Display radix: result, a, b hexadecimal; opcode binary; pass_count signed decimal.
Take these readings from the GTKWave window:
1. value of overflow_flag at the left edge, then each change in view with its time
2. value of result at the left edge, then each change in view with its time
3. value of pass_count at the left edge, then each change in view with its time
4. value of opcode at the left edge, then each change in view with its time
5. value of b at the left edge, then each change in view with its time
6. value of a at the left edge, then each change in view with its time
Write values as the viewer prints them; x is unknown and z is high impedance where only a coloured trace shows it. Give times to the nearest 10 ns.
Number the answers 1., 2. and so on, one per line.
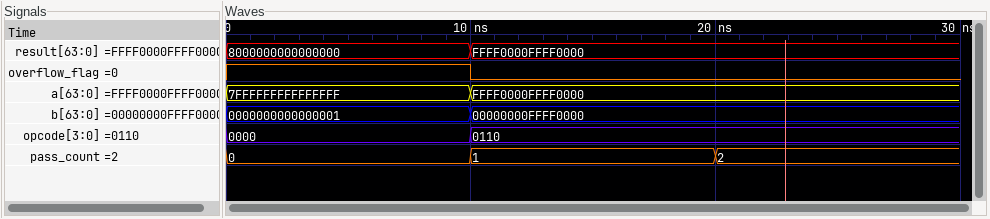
1. 1, 0 at 10 ns
2. 8000000000000000, FFFF0000FFFF0000 at 10 ns
3. 0, 1 at 10 ns, 2 at 20 ns
4. 0000, 0110 at 10 ns
5. 0000000000000001, 00000000FFFF0000 at 10 ns
6. 7FFFFFFFFFFFFFFF, FFFF0000FFFF0000 at 10 ns
